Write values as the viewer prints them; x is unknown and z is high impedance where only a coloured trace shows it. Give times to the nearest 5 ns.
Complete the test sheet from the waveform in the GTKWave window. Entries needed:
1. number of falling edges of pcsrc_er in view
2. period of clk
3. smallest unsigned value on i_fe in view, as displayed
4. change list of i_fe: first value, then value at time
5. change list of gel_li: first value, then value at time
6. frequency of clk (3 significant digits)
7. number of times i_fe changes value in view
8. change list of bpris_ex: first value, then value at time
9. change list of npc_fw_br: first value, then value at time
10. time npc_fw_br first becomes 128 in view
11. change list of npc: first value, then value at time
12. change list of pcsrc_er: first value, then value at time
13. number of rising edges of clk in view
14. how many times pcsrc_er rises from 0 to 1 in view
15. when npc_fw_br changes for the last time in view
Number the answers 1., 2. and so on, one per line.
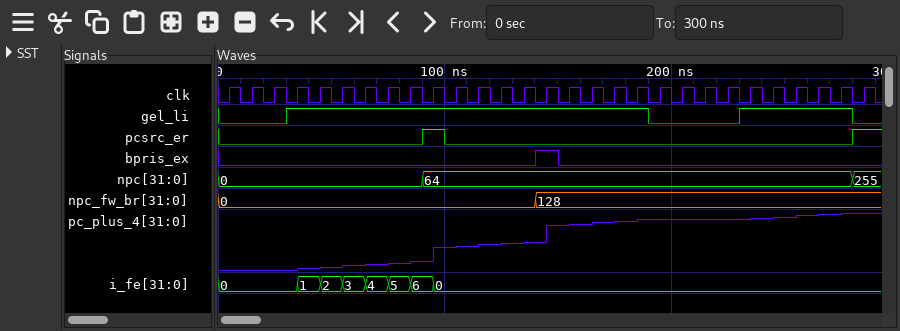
1. 1
2. 10 ns
3. 0
4. 0, 1 at 35 ns, 2 at 45 ns, 3 at 55 ns, 4 at 65 ns, 5 at 75 ns, 6 at 85 ns, 0 at 95 ns
5. 0, 1 at 30 ns, 0 at 190 ns, 1 at 230 ns, 0 at 280 ns
6. 100 MHz
7. 7
8. 0, 1 at 140 ns, 0 at 150 ns
9. 0, 128 at 140 ns
10. 140 ns
11. 0, 64 at 90 ns, 255 at 280 ns
12. 0, 1 at 90 ns, 0 at 100 ns, 1 at 280 ns
13. 29
14. 2
15. 140 ns
